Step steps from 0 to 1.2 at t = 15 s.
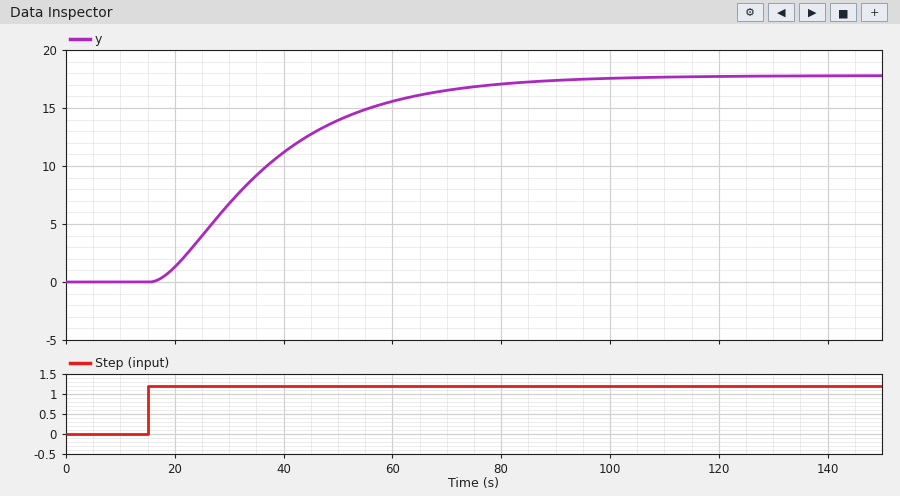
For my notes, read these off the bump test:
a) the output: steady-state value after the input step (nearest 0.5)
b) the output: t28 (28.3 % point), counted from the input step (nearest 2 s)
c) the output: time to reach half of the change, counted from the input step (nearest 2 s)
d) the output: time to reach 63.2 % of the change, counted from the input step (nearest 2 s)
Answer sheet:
18.0
12 s
20 s
26 s
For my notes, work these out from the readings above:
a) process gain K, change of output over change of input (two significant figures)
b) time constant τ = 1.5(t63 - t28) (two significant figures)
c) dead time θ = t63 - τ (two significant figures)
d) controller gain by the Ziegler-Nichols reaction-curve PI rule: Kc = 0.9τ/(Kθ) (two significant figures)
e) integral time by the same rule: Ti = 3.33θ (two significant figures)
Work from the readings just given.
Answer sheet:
15
21 s
5.0 s
0.25
17 s
